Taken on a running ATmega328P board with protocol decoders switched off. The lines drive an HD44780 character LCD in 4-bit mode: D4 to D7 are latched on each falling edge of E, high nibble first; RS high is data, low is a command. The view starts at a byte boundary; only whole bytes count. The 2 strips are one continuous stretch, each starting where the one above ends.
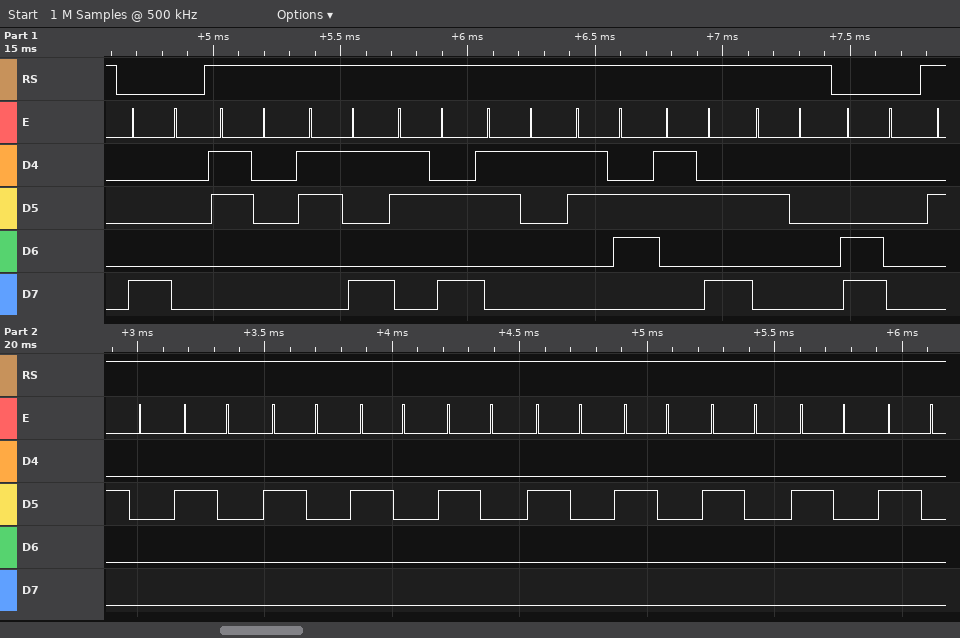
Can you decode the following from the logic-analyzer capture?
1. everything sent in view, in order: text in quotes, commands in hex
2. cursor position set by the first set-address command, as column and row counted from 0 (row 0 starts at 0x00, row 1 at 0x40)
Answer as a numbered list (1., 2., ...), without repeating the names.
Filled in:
1. 0x80 "09:16: " 0xC0 "          "
2. column 0, row 0
